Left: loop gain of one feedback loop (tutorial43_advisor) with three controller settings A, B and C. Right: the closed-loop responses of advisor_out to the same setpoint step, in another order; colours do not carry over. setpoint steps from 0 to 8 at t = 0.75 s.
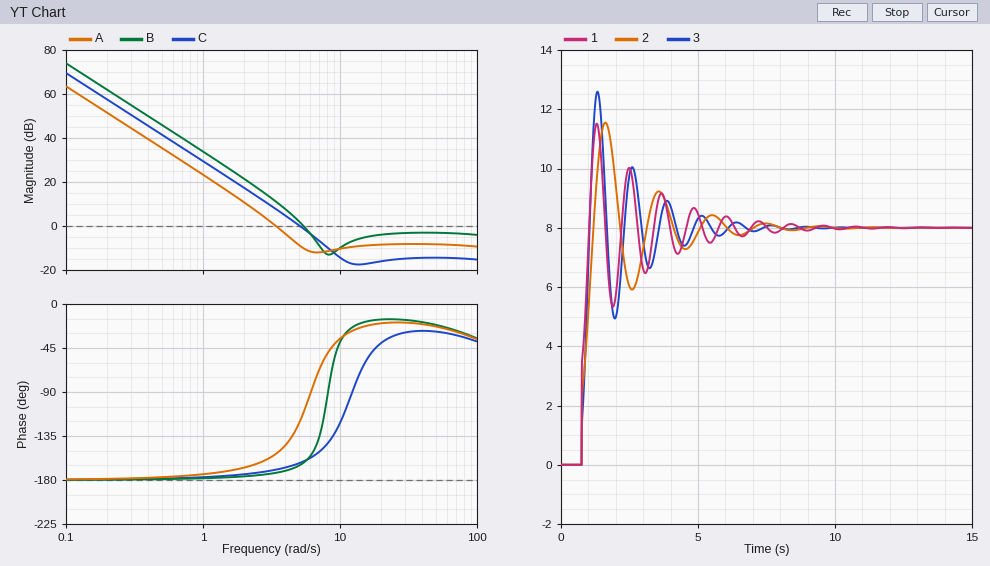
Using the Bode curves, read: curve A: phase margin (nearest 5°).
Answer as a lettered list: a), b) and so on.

a) 25°
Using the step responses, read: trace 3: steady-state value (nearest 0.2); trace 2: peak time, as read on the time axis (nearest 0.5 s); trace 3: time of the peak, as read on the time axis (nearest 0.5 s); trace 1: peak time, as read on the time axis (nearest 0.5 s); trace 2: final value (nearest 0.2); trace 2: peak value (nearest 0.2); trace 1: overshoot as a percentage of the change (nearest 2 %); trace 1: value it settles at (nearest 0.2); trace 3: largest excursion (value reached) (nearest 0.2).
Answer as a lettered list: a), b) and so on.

a) 8.0
b) 1.5 s
c) 1.5 s
d) 1.5 s
e) 8.0
f) 11.6
g) 44 %
h) 8.0
i) 12.6
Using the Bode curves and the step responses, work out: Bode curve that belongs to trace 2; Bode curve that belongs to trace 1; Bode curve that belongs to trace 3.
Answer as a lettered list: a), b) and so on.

a) A
b) B
c) C
